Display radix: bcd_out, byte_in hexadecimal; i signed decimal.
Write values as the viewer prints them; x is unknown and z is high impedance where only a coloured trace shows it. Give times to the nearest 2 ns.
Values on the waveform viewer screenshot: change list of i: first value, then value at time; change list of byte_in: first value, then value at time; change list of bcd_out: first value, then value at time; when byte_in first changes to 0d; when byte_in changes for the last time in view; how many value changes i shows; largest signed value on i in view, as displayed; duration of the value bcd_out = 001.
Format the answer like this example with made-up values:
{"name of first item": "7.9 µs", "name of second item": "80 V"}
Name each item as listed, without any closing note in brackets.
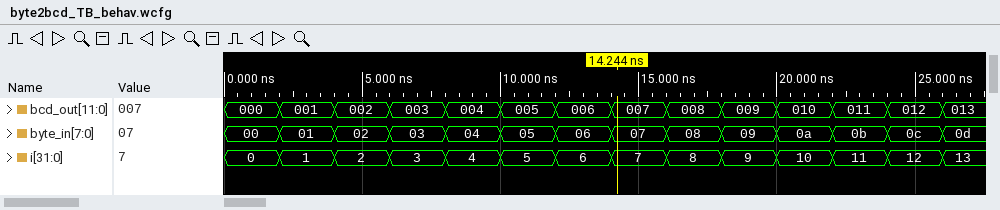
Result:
{"change list of i: first value, then value at time": "0, 1 at 2 ns, 2 at 4 ns, 3 at 6 ns, 4 at 8 ns, 5 at 10 ns, 6 at 12 ns, 7 at 14 ns, 8 at 16 ns, 9 at 18 ns, 10 at 20 ns, 11 at 22 ns, 12 at 24 ns, 13 at 26 ns", "change list of byte_in: first value, then value at time": "00, 01 at 2 ns, 02 at 4 ns, 03 at 6 ns, 04 at 8 ns, 05 at 10 ns, 06 at 12 ns, 07 at 14 ns, 08 at 16 ns, 09 at 18 ns, 0a at 20 ns, 0b at 22 ns, 0c at 24 ns, 0d at 26 ns", "change list of bcd_out: first value, then value at time": "000, 001 at 2 ns, 002 at 4 ns, 003 at 6 ns, 004 at 8 ns, 005 at 10 ns, 006 at 12 ns, 007 at 14 ns, 008 at 16 ns, 009 at 18 ns, 010 at 20 ns, 011 at 22 ns, 012 at 24 ns, 013 at 26 ns", "when byte_in first changes to 0d": "26 ns", "when byte_in changes for the last time in view": "26 ns", "how many value changes i shows": "13", "largest signed value on i in view, as displayed": "13", "duration of the value bcd_out = 001": "2 ns"}
